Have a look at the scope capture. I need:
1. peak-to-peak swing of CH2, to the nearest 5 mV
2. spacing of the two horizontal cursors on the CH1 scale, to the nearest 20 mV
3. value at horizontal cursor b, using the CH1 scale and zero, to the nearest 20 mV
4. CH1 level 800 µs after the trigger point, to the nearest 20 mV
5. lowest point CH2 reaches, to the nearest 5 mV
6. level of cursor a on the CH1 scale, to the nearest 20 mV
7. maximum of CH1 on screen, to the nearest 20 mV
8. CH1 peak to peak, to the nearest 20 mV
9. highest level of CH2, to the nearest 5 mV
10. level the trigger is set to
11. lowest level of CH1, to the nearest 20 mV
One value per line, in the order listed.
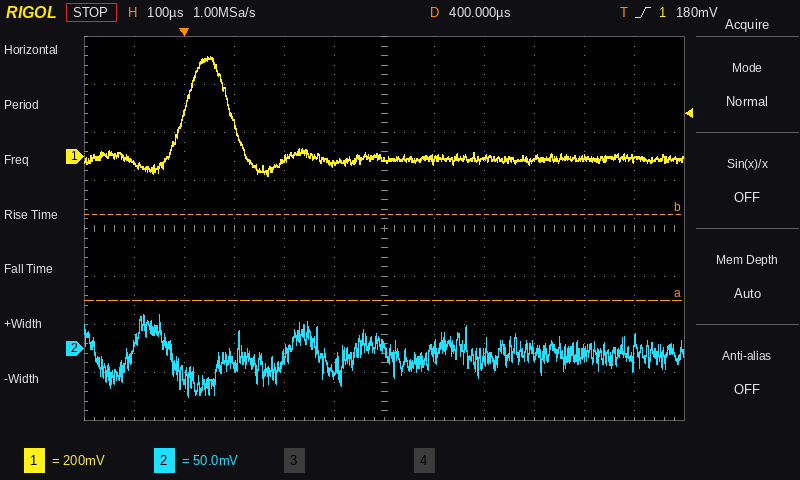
85 mV
360 mV
-240 mV
0 mV
-50 mV
-600 mV
420 mV
500 mV
35 mV
180 mV
-80 mV
